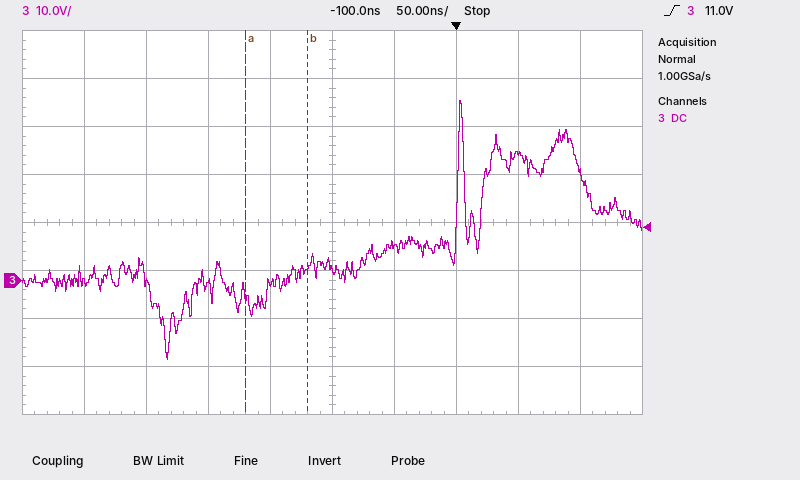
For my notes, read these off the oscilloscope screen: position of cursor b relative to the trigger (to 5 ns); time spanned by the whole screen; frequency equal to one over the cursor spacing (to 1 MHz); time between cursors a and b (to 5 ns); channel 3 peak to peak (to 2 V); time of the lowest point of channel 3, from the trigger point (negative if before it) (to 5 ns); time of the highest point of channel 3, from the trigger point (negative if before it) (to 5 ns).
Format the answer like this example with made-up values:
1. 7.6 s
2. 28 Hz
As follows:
1. -120 ns
2. 500 ns
3. 20 MHz
4. 50 ns
5. 54 V
6. -235 ns
7. +5 ns
